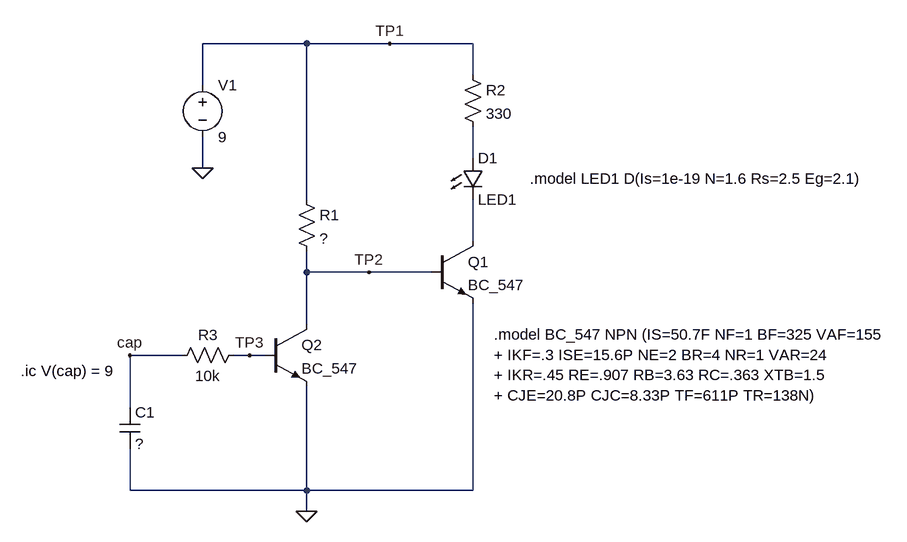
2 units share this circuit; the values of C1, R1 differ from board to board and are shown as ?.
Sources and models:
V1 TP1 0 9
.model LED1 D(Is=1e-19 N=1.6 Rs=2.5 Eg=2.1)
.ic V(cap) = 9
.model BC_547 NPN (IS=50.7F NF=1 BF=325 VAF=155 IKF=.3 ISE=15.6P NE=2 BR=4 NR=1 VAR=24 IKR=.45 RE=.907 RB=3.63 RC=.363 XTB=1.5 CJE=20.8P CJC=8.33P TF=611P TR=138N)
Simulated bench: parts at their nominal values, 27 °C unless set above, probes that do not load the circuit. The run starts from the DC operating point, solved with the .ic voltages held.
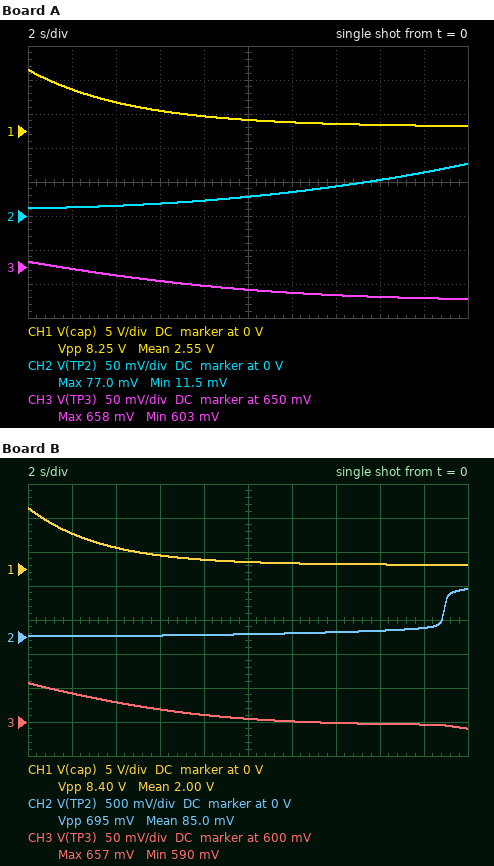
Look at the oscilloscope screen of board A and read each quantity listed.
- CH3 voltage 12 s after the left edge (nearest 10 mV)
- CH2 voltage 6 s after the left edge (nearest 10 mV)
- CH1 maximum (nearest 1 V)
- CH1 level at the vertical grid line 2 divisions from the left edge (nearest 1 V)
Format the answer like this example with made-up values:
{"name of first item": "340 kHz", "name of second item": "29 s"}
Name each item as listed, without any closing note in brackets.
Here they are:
{"CH3 voltage 12 s after the left edge": "610 mV", "CH2 voltage 6 s after the left edge": "20 mV", "CH1 maximum": "9 V", "CH1 level at the vertical grid line 2 divisions from the left edge": "4 V"}
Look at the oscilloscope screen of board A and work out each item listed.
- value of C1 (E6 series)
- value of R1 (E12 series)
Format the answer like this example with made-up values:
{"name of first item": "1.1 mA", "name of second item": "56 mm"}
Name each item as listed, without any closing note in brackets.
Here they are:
{"value of C1": "470 µF", "value of R1": "15 kΩ"}
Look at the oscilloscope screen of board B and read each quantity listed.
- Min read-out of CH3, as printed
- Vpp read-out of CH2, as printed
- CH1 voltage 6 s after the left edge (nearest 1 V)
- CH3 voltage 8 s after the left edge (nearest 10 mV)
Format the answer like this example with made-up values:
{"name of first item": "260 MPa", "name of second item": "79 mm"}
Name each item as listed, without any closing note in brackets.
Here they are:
{"Min read-out of CH3, as printed": "590 mV", "Vpp read-out of CH2, as printed": "695 mV", "CH1 voltage 6 s after the left edge": "2 V", "CH3 voltage 8 s after the left edge": "610 mV"}
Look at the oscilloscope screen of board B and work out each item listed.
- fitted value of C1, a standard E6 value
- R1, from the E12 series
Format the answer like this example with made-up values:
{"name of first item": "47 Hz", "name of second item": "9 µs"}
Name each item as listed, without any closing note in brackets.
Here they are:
{"fitted value of C1, a standard E6 value": "330 µF", "R1, from the E12 series": "18 kΩ"}
